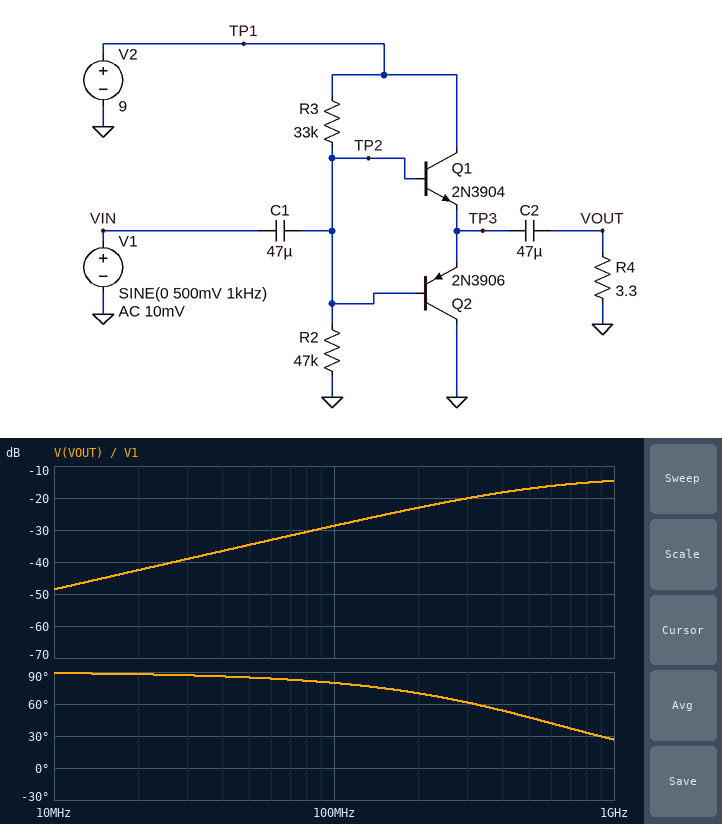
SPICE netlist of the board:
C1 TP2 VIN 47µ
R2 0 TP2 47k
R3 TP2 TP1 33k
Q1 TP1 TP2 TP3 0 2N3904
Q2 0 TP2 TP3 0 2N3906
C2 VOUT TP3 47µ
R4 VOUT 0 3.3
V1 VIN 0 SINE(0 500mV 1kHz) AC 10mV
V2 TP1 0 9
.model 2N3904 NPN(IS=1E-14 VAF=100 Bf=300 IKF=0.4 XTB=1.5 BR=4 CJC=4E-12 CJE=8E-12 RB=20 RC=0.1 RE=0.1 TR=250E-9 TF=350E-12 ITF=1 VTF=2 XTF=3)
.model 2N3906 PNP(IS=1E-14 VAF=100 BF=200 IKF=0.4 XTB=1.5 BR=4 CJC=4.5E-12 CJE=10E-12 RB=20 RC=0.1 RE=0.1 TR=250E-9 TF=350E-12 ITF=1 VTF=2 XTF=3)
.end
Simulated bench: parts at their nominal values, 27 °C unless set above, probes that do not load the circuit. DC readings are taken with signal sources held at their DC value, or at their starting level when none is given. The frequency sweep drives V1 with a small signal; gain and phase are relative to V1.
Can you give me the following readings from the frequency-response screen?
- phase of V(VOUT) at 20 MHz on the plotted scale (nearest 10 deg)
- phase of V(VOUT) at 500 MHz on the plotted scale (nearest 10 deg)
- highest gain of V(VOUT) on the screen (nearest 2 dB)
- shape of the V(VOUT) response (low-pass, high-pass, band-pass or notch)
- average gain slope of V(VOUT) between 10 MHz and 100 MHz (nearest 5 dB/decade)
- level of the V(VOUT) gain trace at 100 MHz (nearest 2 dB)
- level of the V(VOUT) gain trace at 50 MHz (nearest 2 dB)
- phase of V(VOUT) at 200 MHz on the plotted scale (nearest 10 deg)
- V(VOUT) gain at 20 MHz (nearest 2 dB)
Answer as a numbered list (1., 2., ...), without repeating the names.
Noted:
1. 90 deg
2. 50 deg
3. -14 dB
4. high-pass
5. 20 dB/decade
6. -28 dB
7. -34 dB
8. 70 deg
9. -42 dB
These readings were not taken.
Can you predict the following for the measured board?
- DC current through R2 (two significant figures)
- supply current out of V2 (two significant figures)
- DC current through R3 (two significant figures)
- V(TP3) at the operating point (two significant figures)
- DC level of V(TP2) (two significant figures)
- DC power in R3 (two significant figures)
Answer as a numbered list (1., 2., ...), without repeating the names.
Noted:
1. 110 µA
2. 110 µA
3. 110 µA
4. 5.3 V
5. 5.3 V
6. 420 µW
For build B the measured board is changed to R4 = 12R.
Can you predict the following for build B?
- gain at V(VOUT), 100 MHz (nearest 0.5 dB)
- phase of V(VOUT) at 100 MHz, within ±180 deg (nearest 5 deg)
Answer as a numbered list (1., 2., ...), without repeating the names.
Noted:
1. -17.5 dB
2. 75 deg
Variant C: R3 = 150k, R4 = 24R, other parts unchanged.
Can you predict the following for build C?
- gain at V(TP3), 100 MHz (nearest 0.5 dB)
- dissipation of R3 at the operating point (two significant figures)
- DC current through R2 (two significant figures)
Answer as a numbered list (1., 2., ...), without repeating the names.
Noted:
1. -12.0 dB
2. 310 µW
3. 46 µA
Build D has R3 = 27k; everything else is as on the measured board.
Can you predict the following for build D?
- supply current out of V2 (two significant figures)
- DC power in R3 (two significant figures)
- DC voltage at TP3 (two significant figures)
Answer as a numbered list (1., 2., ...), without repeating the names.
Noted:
1. 120 µA
2. 400 µW
3. 5.7 V
